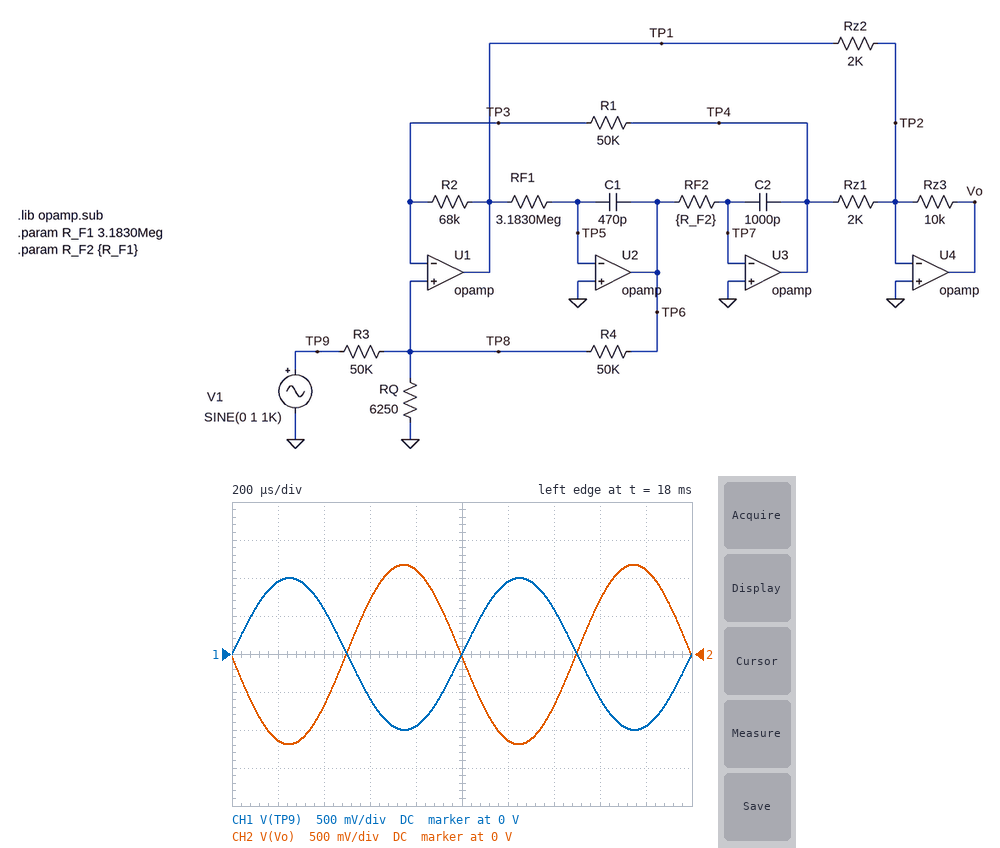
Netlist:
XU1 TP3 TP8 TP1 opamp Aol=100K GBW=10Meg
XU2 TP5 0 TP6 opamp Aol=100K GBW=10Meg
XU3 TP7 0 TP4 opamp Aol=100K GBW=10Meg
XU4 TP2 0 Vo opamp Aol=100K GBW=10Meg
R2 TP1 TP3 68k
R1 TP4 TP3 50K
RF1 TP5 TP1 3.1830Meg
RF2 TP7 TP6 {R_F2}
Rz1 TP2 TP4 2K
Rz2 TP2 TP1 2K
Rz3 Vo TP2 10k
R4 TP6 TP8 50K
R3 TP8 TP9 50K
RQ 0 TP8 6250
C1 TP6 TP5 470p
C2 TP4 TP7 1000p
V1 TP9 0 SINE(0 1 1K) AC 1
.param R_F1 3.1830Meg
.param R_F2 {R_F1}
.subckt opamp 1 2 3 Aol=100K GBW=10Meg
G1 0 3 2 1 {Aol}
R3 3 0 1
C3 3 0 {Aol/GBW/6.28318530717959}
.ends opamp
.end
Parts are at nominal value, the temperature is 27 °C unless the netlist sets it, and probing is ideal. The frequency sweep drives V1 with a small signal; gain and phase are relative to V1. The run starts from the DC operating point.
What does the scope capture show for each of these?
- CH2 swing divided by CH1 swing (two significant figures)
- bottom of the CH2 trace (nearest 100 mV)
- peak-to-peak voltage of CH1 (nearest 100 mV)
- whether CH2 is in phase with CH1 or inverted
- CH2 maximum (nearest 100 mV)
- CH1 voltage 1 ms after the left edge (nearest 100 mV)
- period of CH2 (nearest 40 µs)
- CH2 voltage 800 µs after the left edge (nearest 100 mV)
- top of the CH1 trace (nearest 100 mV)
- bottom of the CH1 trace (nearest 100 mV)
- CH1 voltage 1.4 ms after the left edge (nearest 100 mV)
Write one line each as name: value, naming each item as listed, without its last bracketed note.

CH2 swing divided by CH1 swing: 1.2
bottom of the CH2 trace: -1.2 V
peak-to-peak voltage of CH1: 2.0 V
whether CH2 is in phase with CH1 or inverted: inverted
CH2 maximum: 1.2 V
CH1 voltage 1 ms after the left edge: 0 V
period of CH2: 1.00 ms
CH2 voltage 800 µs after the left edge: 1.1 V
top of the CH1 trace: 1.0 V
bottom of the CH1 trace: -1.0 V
CH1 voltage 1.4 ms after the left edge: 600 mV
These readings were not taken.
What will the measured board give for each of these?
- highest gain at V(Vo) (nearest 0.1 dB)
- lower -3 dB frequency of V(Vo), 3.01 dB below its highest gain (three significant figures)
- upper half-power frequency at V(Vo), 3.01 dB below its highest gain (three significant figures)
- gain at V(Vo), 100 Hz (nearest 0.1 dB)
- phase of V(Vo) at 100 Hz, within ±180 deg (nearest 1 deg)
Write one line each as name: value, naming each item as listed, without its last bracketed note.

highest gain at V(Vo): 3.4 dB
lower -3 dB frequency of V(Vo), 3.01 dB below its highest gain: 84.9 Hz
upper half-power frequency at V(Vo), 3.01 dB below its highest gain: 460 kHz
gain at V(Vo), 100 Hz: 3.4 dB
phase of V(Vo) at 100 Hz, within ±180 deg: -138 deg
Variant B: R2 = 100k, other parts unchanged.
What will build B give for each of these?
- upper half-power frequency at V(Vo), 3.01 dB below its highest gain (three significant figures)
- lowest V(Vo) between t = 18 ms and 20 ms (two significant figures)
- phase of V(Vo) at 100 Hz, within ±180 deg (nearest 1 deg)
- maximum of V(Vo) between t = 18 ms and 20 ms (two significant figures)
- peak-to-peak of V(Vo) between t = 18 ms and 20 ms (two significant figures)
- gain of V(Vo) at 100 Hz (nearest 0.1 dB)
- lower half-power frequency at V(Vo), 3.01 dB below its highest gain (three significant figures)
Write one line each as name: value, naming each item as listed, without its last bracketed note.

upper half-power frequency at V(Vo), 3.01 dB below its highest gain: 164 Hz
lowest V(Vo) between t = 18 ms and 20 ms: -1.5 V
phase of V(Vo) at 100 Hz, within ±180 deg: -79 deg
maximum of V(Vo) between t = 18 ms and 20 ms: 1.5 V
peak-to-peak of V(Vo) between t = 18 ms and 20 ms: 3.0 V
gain of V(Vo) at 100 Hz: 6.7 dB
lower half-power frequency at V(Vo), 3.01 dB below its highest gain: 97.5 Hz
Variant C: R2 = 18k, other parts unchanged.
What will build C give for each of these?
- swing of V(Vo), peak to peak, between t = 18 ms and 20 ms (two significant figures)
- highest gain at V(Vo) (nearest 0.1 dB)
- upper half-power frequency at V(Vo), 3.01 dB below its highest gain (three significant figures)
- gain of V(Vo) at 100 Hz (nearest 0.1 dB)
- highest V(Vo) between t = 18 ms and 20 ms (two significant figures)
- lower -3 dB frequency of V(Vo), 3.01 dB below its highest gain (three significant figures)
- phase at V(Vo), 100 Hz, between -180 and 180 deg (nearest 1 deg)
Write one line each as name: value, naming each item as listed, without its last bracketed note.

swing of V(Vo), peak to peak, between t = 18 ms and 20 ms: 1.4 V
highest gain at V(Vo): 11.8 dB
upper half-power frequency at V(Vo), 3.01 dB below its highest gain: 47.4 Hz
gain of V(Vo) at 100 Hz: -8.2 dB
highest V(Vo) between t = 18 ms and 20 ms: 700 mV
lower -3 dB frequency of V(Vo), 3.01 dB below its highest gain: 30.3 Hz
phase at V(Vo), 100 Hz, between -180 and 180 deg: -170 deg
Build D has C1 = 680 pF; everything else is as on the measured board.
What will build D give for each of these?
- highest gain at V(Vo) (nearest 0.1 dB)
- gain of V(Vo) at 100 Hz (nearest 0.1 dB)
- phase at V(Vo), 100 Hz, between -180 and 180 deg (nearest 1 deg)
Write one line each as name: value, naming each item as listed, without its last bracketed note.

highest gain at V(Vo): 4.3 dB
gain of V(Vo) at 100 Hz: 3.0 dB
phase at V(Vo), 100 Hz, between -180 and 180 deg: -161 deg
